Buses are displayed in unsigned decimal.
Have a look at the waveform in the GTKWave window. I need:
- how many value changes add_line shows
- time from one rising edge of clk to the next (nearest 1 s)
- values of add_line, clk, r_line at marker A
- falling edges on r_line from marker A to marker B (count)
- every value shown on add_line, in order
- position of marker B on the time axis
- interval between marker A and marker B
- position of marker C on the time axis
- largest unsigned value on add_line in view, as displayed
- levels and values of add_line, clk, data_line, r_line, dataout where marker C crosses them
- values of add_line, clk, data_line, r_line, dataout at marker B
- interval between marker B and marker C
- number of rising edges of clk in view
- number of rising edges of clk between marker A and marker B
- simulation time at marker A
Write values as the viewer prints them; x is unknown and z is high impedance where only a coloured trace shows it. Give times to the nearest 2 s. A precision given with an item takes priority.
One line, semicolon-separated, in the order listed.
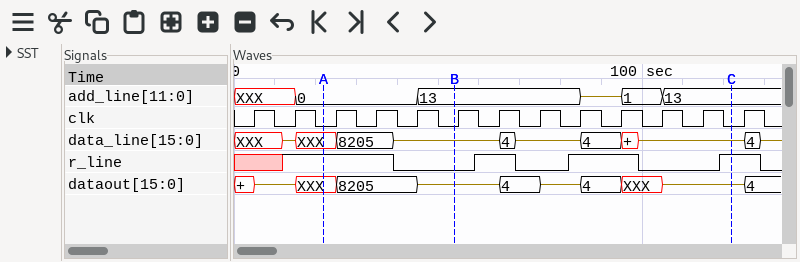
5; 10 s; add_line=0, clk=0, r_line=1; 1; XXX, 0, 13, z, 1, 13; 54 s; 32 s; 122 s; 13; add_line=13, clk=0, data_line=z, r_line=1, dataout=z; add_line=13, clk=0, data_line=z, r_line=0, dataout=z; 68 s; 13; 3; 22 s
